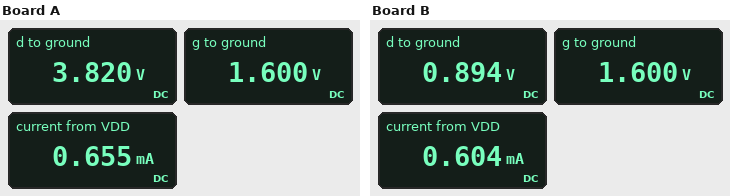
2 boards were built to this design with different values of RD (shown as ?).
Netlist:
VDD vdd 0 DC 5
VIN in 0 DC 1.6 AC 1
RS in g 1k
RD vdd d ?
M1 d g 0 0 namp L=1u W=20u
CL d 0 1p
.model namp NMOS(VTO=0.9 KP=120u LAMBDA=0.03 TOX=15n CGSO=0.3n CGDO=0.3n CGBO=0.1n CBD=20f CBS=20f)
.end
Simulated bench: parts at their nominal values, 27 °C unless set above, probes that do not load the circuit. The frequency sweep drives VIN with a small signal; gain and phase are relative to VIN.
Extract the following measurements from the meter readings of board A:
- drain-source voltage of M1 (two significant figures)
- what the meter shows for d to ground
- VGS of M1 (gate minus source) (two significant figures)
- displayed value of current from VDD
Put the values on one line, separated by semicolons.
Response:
3.8 V; 3.820 V; 1.6 V; 0.655 mA
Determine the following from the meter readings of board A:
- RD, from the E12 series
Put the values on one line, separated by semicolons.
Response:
1.8 kΩ
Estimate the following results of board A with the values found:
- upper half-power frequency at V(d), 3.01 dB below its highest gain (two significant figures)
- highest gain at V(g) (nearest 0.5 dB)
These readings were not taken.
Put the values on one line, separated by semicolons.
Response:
89 MHz; 0 dB
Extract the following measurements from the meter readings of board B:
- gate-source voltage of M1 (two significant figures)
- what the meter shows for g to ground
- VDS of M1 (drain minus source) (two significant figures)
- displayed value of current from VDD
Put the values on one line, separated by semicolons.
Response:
1.6 V; 1.600 V; 890 mV; 0.604 mA
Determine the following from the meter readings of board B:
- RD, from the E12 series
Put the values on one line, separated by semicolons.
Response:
6.8 kΩ
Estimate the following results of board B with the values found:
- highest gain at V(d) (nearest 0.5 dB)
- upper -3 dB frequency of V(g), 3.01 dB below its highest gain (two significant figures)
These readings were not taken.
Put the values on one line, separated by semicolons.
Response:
20.5 dB; 3.7 GHz
